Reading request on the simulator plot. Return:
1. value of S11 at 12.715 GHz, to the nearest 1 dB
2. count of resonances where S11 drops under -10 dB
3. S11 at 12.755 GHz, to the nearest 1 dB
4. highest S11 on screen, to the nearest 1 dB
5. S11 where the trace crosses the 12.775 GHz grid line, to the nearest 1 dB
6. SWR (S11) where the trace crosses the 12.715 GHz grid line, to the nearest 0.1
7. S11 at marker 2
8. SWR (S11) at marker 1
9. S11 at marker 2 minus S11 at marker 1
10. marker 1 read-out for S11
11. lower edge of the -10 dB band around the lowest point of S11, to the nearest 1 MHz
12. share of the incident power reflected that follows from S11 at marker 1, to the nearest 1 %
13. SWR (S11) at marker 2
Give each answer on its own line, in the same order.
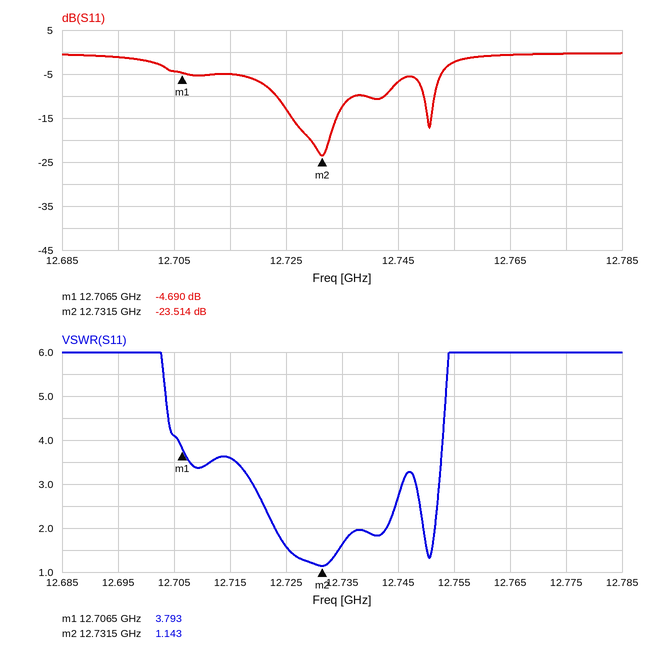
-5 dB
2
-2 dB
0 dB
0 dB
3.6
-23.514 dB
3.793
-18.824 dB
-4.690 dB
12.723 GHz
34 %
1.143
